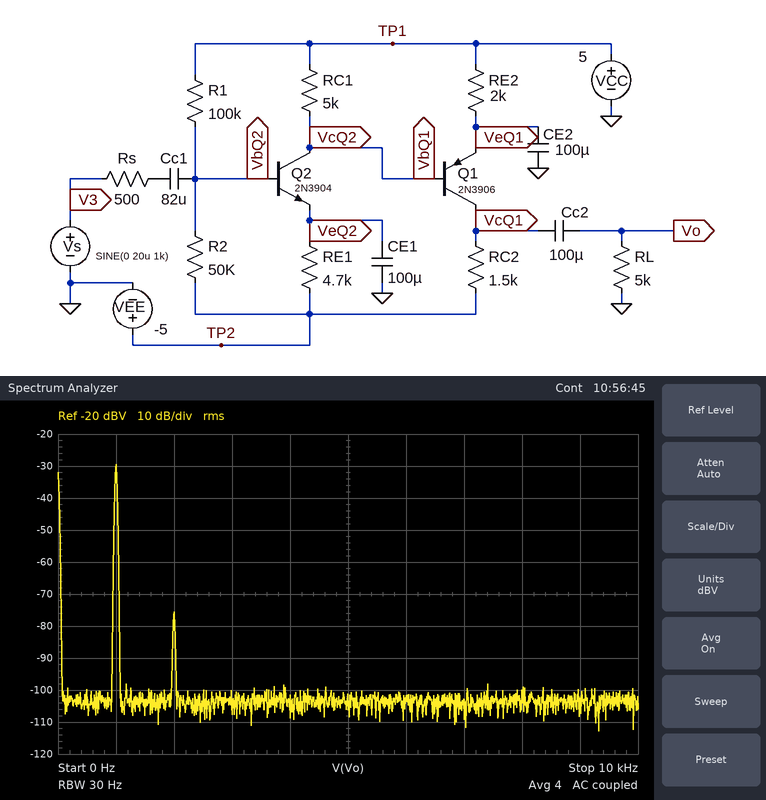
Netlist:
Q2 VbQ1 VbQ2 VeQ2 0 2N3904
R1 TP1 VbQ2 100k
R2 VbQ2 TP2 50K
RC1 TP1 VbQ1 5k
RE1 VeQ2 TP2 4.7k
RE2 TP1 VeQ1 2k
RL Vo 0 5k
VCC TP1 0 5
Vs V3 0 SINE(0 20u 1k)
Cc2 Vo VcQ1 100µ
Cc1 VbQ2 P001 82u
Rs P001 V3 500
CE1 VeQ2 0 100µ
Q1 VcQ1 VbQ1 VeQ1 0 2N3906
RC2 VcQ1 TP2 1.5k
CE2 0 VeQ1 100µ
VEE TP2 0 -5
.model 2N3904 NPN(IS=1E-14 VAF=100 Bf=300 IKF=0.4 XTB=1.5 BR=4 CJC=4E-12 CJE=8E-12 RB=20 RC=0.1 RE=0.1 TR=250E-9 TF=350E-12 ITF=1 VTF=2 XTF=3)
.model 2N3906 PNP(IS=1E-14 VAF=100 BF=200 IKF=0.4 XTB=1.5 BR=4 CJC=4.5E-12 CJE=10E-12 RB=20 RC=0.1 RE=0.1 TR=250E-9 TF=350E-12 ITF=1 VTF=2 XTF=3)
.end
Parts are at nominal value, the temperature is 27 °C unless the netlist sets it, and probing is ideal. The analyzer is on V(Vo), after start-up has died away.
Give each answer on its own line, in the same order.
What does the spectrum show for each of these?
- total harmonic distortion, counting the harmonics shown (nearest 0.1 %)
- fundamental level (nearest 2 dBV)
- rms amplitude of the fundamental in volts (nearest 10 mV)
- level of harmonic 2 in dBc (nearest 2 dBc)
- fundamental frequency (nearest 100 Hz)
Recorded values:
0.5 %
-30 dBV
30 mV
-46 dBc
1.0 kHz
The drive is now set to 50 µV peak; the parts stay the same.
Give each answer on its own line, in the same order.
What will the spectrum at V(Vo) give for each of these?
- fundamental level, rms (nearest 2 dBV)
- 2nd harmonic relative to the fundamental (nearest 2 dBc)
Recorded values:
-22 dBV
-38 dBc
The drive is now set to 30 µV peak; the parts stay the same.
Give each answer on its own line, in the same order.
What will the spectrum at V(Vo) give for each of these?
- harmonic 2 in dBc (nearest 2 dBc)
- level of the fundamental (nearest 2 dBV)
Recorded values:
-42 dBc
-26 dBV
